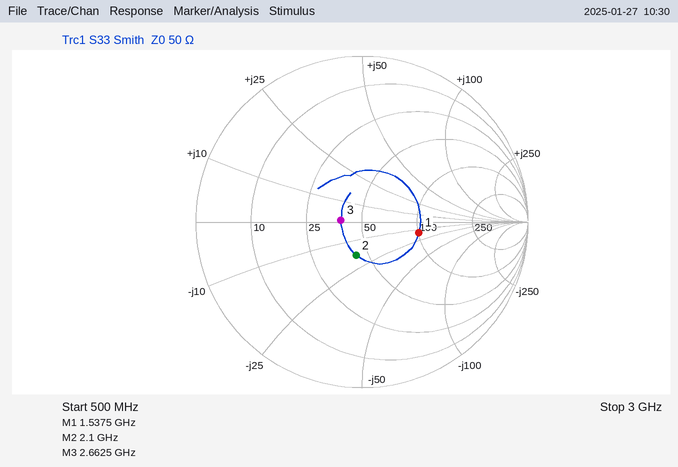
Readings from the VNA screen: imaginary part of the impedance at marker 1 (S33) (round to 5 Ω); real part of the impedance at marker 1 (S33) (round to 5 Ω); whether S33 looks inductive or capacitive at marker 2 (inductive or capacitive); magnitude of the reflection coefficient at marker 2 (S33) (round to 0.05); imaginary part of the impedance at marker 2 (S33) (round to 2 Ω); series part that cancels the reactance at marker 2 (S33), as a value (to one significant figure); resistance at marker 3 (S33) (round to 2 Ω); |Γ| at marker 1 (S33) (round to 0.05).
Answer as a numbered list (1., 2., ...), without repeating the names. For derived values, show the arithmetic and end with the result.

1. -15 Ω
2. 100 Ω
3. capacitive
4. 0.20
5. -18 Ω
6. L = 18 Ω/(2π × 2.1 GHz) ≈ 1 nH
7. 38 Ω
8. 0.35
